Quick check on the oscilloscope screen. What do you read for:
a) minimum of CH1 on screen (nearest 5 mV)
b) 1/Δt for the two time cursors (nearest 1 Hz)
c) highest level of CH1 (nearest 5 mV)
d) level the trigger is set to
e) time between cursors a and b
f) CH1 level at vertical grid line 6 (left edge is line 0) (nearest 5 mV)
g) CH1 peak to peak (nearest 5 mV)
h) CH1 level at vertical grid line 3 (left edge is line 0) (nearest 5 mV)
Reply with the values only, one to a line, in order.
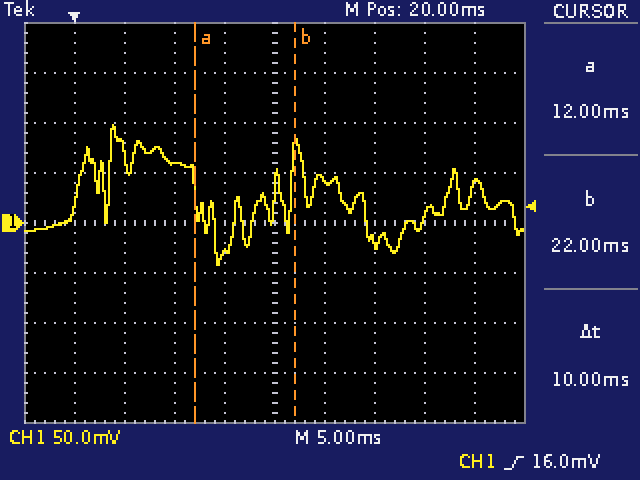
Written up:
-40 mV
100 Hz
100 mV
16.0 mV
10 ms
45 mV
140 mV
60 mV
